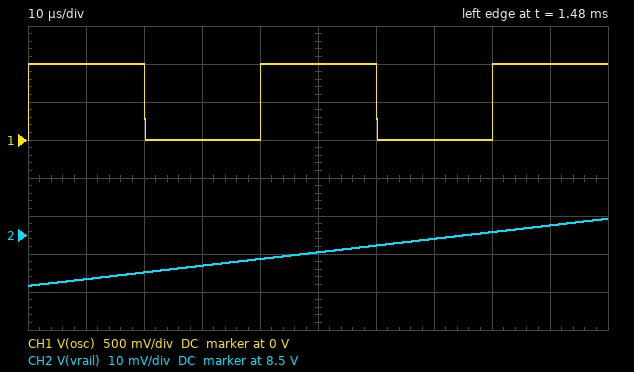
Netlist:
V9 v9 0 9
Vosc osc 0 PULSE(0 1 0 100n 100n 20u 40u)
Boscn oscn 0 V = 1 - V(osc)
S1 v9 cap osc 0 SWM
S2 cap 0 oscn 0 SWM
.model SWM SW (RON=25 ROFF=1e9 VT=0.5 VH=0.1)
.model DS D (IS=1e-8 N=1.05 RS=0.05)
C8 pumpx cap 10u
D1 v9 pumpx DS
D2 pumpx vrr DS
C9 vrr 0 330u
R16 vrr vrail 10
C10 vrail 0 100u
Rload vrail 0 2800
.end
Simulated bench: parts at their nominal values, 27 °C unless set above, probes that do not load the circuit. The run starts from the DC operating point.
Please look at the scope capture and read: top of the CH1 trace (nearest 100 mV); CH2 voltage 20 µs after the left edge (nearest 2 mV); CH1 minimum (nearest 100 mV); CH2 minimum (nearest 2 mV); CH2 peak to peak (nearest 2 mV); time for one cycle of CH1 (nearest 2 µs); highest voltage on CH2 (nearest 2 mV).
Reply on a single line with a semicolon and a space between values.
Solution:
1.0 V; 8.490 V; 0 V; 8.486 V; 18 mV; 40 µs; 8.504 V
